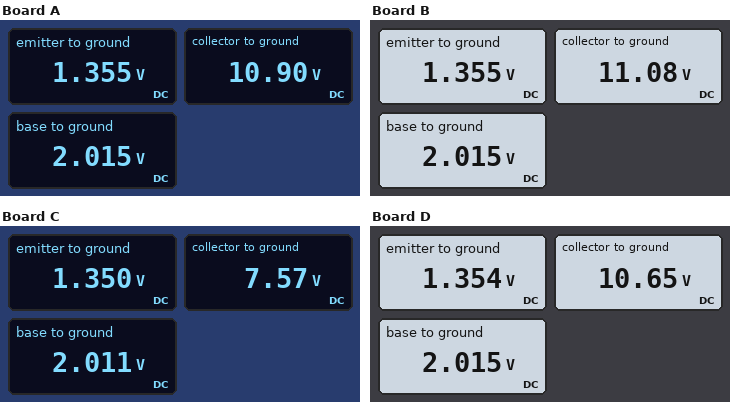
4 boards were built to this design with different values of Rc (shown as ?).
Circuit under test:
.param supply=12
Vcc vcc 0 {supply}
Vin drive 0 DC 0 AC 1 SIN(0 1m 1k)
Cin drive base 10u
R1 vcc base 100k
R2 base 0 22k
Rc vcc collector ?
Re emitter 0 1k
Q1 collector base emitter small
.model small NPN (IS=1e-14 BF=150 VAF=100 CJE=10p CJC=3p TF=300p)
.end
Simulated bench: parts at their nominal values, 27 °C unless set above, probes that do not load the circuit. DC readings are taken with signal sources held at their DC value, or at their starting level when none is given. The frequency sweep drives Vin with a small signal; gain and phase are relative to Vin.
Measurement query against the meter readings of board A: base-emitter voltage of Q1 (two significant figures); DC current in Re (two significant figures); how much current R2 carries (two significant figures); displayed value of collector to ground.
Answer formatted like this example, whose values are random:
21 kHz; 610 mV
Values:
660 mV; 1.4 mA; 92 µA; 10.90 V
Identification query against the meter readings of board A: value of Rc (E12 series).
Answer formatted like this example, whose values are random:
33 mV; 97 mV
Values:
820 Ω
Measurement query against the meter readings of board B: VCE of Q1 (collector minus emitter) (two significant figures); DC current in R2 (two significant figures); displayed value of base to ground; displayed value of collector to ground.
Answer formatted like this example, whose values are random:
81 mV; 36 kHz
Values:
9.7 V; 92 µA; 2.015 V; 11.08 V
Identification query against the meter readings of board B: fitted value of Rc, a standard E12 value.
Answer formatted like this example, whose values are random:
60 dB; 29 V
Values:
680 Ω
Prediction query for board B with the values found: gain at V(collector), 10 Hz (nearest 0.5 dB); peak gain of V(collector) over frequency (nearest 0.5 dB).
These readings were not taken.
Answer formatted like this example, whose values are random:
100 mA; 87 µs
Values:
-3.5 dB; -3.5 dB
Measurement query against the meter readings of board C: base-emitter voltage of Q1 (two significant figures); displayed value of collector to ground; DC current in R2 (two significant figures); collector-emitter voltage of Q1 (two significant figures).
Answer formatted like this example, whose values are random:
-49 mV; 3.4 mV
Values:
660 mV; 7.57 V; 91 µA; 6.2 V
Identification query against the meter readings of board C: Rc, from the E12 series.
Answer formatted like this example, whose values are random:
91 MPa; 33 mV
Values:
3.3 kΩ
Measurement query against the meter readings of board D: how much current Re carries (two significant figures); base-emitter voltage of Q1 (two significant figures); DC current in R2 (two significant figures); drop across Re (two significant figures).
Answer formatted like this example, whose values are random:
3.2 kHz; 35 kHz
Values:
1.4 mA; 660 mV; 92 µA; 1.4 V
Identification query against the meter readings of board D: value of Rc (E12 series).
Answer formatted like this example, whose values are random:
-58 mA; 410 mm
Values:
1 kΩ
